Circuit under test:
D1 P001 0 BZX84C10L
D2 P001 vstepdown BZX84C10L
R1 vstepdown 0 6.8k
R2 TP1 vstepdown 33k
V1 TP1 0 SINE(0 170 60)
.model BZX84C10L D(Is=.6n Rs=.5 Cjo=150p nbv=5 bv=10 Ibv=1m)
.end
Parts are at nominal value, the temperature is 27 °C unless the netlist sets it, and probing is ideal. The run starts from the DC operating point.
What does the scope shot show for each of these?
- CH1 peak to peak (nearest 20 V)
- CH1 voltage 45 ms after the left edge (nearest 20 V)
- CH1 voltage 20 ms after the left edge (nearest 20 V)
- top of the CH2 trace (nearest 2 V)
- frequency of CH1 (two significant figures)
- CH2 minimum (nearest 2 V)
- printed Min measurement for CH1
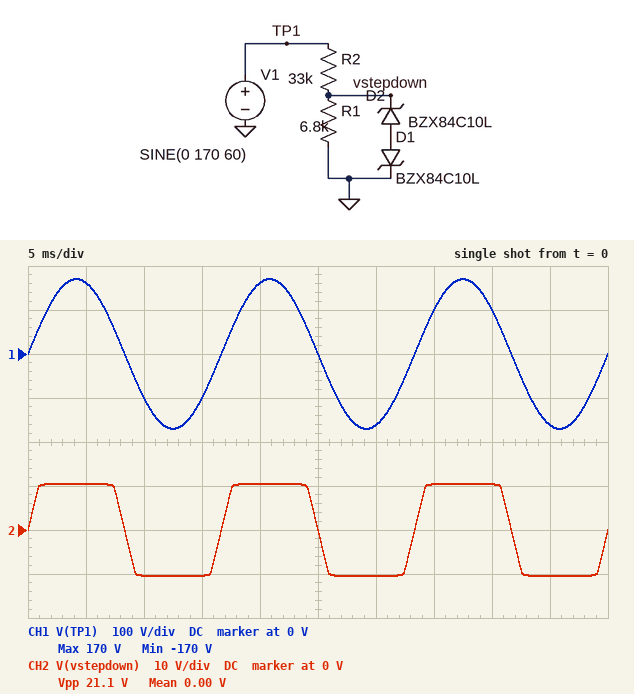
340 V
-160 V
160 V
10 V
60 Hz
-10 V
-170 V
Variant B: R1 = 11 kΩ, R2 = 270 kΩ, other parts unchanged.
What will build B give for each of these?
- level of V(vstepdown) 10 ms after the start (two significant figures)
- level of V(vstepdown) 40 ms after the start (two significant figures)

-3.9 V
3.9 V
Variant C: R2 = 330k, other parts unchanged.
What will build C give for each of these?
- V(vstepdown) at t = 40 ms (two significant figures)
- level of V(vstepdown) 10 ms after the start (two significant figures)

2.0 V
-2.0 V
